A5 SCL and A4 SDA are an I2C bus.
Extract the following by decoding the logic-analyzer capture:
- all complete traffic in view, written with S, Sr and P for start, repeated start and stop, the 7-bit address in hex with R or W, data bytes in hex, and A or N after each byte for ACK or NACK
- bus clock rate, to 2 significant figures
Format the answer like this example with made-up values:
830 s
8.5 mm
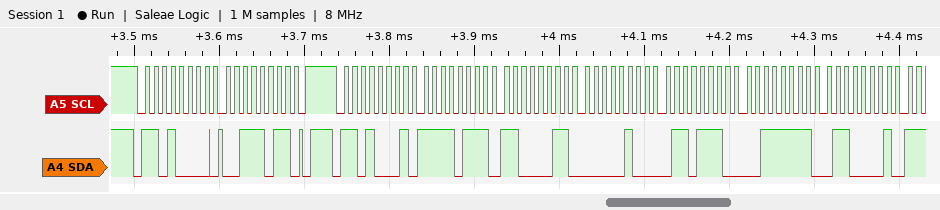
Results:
S 68W A 3B A P S 68R A F7 A C3 A 04 A 6E A 3F A 61 A
100 kHz
